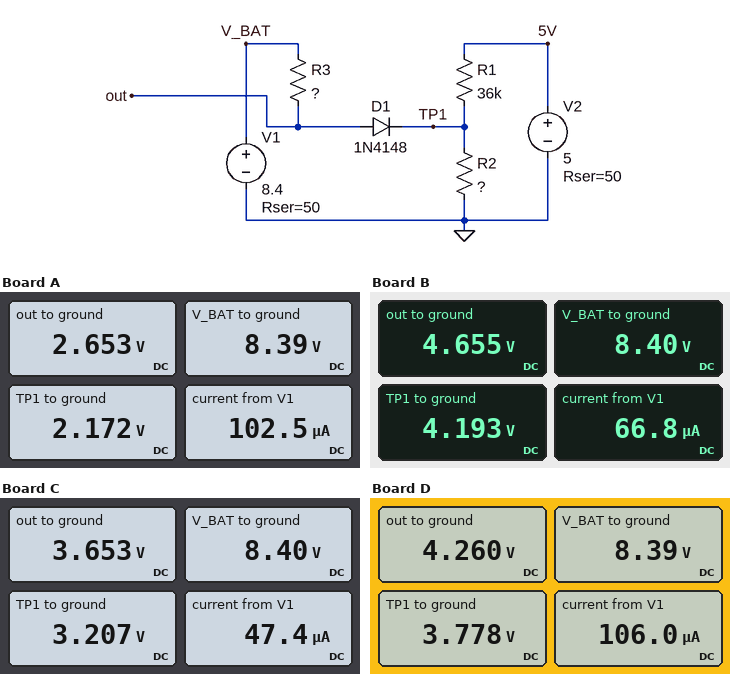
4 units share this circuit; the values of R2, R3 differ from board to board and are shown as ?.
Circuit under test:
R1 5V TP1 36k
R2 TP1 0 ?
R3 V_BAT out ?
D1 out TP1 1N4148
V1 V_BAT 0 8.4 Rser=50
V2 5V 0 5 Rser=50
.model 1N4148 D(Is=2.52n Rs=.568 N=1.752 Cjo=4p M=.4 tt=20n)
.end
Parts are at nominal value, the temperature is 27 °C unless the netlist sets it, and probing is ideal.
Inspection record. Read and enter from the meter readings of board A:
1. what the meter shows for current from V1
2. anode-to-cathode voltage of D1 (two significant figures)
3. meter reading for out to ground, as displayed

102.5 µA
480 mV
2.653 V
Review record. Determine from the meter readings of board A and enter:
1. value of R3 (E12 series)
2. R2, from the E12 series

56 kΩ
12 kΩ
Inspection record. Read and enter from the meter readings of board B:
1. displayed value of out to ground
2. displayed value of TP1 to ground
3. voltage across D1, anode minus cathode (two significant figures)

4.655 V
4.193 V
460 mV
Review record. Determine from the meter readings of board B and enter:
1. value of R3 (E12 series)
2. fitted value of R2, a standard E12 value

56 kΩ
47 kΩ
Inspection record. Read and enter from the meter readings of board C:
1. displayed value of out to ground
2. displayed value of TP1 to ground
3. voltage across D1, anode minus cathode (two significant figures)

3.653 V
3.207 V
450 mV
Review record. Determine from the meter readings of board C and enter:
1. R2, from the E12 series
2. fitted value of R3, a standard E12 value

33 kΩ
100 kΩ
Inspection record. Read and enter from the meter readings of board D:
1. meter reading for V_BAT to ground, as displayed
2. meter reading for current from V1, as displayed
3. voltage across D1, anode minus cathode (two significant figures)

8.39 V
106.0 µA
480 mV
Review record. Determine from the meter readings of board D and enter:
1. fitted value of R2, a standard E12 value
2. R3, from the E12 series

27 kΩ
39 kΩ
